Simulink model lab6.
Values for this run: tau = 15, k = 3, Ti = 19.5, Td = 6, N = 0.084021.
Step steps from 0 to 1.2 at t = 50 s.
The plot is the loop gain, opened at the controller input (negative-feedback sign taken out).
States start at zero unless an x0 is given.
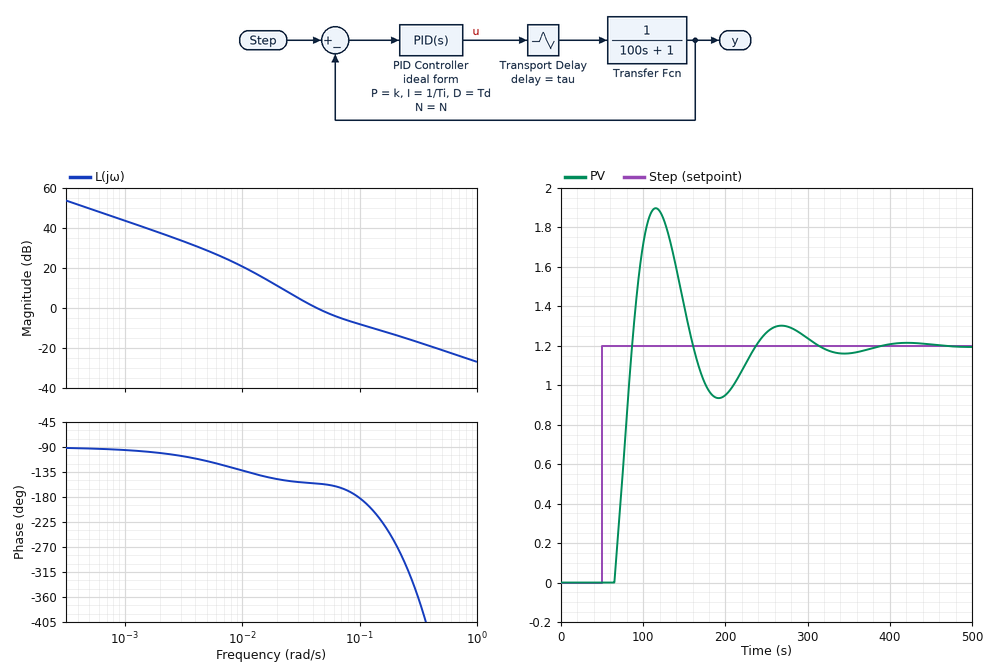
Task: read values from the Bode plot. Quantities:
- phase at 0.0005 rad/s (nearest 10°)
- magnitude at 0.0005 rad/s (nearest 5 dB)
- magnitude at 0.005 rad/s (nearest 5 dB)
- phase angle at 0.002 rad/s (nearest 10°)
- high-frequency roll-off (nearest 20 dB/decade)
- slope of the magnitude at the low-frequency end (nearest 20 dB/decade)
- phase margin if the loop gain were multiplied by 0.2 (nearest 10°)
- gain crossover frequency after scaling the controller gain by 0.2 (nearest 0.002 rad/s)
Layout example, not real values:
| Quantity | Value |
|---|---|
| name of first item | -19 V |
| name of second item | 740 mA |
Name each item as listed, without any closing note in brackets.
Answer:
| Quantity | Value |
|---|---|
| phase at 0.0005 rad/s | -90° |
| magnitude at 0.0005 rad/s | 50 dB |
| magnitude at 0.005 rad/s | 30 dB |
| phase angle at 0.002 rad/s | -100° |
| high-frequency roll-off | -20 dB/decade |
| slope of the magnitude at the low-frequency end | -20 dB/decade |
| phase margin if the loop gain were multiplied by 0.2 | 40° |
| gain crossover frequency after scaling the controller gain by 0.2 | 0.016 rad/s |
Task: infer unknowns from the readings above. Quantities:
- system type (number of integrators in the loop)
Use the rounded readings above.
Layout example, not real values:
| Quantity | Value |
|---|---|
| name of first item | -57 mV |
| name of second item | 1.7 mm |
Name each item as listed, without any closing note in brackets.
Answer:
| Quantity | Value |
|---|---|
| system type | 1 |
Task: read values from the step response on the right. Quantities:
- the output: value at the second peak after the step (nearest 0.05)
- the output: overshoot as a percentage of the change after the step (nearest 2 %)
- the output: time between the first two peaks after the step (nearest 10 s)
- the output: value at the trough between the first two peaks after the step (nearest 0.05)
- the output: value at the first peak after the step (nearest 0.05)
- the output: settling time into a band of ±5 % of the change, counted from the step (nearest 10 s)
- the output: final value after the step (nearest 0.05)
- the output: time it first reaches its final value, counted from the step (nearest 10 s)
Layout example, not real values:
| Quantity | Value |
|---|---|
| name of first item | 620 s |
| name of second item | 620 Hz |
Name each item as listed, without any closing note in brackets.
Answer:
| Quantity | Value |
|---|---|
| the output: value at the second peak after the step | 1.30 |
| the output: overshoot as a percentage of the change after the step | 58 % |
| the output: time between the first two peaks after the step | 150 s |
| the output: value at the trough between the first two peaks after the step | 0.95 |
| the output: value at the first peak after the step | 1.90 |
| the output: settling time into a band of ±5 % of the change, counted from the step | 240 s |
| the output: final value after the step | 1.20 |
| the output: time it first reaches its final value, counted from the step | 40 s |
